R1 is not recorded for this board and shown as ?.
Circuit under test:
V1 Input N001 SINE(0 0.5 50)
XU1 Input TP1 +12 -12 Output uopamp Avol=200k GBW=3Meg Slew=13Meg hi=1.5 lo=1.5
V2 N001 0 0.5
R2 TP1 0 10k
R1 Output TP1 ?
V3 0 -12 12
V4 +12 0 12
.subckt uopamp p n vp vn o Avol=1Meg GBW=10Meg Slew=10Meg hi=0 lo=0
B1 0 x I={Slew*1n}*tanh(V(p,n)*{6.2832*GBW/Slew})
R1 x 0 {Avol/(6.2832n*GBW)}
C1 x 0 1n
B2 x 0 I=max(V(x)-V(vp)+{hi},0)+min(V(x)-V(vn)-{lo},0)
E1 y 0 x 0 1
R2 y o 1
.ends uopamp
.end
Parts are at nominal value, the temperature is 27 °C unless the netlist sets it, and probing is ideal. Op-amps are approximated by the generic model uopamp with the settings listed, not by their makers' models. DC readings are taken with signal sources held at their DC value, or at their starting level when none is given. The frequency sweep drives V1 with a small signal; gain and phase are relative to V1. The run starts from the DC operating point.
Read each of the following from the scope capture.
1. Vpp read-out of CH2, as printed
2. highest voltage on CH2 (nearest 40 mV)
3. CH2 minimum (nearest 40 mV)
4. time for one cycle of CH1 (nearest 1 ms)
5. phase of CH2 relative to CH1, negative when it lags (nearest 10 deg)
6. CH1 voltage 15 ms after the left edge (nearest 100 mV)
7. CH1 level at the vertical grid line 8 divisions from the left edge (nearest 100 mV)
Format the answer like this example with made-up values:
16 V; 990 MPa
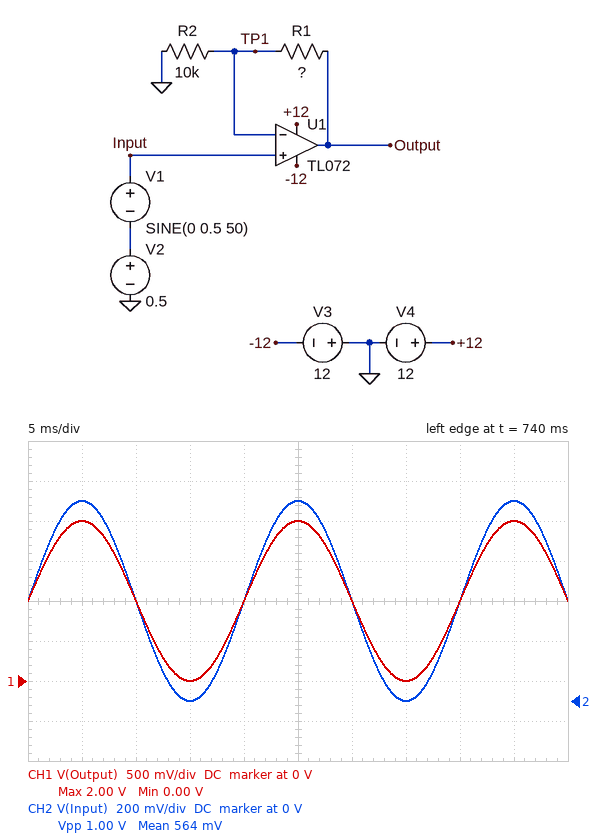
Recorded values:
1.00 V; 1.00 V; 0 V; 20 ms; 0 deg; 0 V; 1.0 V
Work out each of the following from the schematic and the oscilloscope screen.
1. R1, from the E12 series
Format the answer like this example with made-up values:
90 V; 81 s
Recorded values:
10 kΩ
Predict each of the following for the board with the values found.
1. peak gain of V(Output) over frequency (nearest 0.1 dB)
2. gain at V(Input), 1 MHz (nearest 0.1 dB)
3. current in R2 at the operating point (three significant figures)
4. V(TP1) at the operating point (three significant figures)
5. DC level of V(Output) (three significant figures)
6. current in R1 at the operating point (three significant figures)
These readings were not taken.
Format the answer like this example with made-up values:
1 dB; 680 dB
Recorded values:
6.0 dB; 0 dB; 50.0 µA; 500 mV; 1.00 V; 50.0 µA
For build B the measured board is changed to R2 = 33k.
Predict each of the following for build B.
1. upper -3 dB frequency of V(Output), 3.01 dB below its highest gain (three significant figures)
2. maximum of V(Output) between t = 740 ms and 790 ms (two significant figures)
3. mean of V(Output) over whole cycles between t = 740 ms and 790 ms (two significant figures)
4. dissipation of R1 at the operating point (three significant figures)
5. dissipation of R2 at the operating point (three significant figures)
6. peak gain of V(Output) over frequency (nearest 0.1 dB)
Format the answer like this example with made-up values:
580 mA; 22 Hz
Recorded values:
2.30 MHz; 1.3 V; 650 mV; 2.30 µW; 7.58 µW; 2.3 dB
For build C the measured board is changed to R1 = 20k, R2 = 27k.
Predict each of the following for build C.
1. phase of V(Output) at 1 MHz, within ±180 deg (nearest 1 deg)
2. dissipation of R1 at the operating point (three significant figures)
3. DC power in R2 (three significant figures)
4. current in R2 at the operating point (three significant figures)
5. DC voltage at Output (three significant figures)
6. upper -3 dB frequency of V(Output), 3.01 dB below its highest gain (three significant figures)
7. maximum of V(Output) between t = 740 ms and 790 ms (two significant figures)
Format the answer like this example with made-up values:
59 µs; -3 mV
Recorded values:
-30 deg; 6.86 µW; 9.26 µW; 18.5 µA; 870 mV; 1.72 MHz; 1.7 V
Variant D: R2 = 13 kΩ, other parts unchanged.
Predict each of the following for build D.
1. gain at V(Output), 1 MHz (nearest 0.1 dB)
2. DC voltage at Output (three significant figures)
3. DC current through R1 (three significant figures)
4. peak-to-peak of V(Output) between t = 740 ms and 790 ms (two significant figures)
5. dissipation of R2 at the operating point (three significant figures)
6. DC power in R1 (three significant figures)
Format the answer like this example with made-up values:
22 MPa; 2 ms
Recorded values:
3.7 dB; 885 mV; 38.5 µA; 1.8 V; 19.2 µW; 14.8 µW
